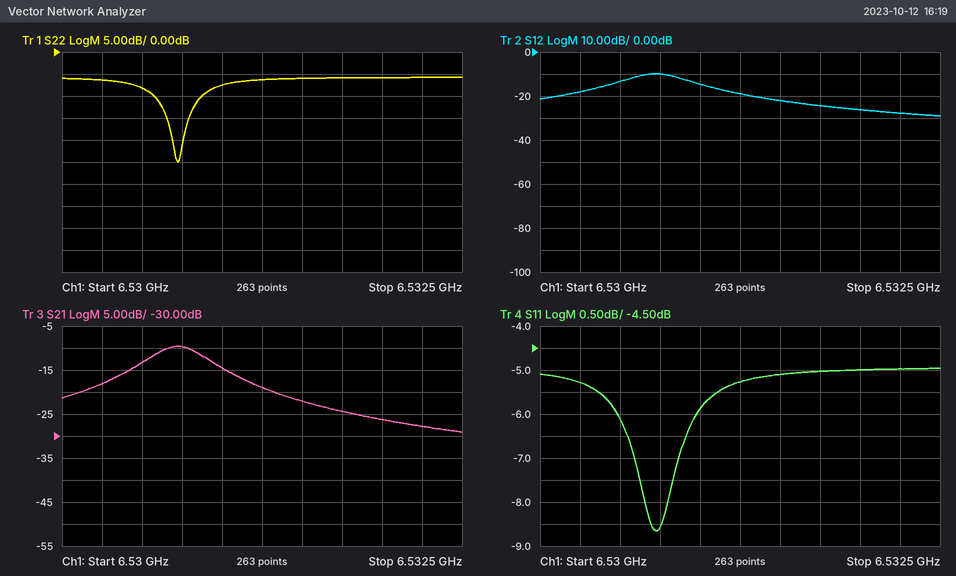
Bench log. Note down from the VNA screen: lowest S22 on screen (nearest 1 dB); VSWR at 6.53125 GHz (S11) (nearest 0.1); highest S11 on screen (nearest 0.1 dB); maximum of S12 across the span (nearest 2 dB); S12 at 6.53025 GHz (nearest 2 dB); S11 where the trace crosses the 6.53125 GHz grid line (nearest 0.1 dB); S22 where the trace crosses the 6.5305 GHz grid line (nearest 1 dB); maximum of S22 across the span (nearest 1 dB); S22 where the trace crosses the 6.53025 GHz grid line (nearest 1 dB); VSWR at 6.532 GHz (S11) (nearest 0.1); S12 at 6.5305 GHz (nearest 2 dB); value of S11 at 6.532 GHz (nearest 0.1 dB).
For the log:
-25 dB
3.4
-5.0 dB
-10 dB
-18 dB
-5.3 dB
-8 dB
-6 dB
-6 dB
3.6
-14 dB
-5.0 dB
